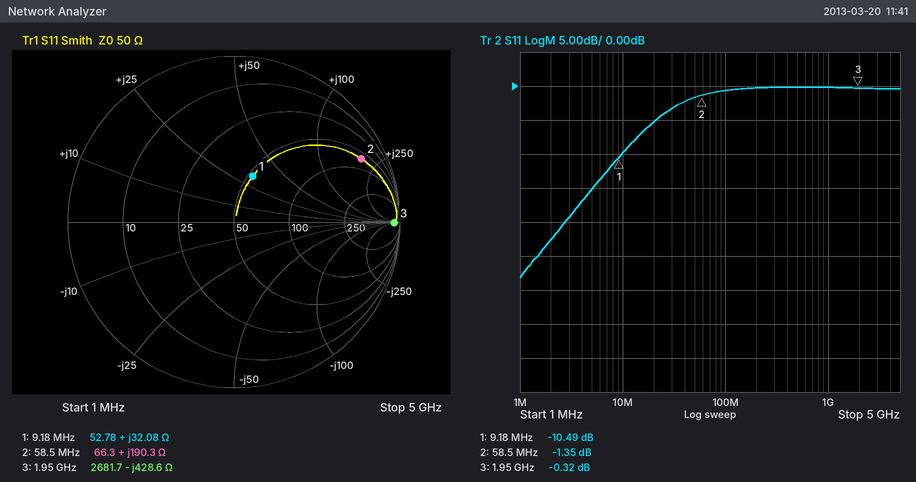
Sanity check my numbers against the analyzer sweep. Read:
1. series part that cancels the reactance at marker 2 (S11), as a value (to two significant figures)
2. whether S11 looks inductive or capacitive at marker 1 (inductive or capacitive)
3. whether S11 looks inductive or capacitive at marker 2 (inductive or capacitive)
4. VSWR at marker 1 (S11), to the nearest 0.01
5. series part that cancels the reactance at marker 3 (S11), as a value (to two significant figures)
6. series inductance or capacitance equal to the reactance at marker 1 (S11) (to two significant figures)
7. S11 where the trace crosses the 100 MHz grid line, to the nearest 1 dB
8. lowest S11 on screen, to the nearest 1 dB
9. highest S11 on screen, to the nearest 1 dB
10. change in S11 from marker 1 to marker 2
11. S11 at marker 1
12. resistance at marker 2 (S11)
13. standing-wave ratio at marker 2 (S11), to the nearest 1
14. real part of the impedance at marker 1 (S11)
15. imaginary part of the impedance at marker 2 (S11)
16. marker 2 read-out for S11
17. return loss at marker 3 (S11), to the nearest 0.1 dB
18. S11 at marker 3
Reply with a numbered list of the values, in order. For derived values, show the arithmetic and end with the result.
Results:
1. C = 1/(2π × 58.5 MHz × 190.3 Ω) ≈ 14 pF
2. inductive
3. inductive
4. 1.85
5. L = 428.6 Ω/(2π × 1.95 GHz) ≈ 35 nH
6. L = 32.08 Ω/(2π × 9.18 MHz) ≈ 556 nH, so 560 nH to two significant figures
7. -1 dB
8. -28 dB
9. 0 dB
10. -1.35 − (-10.49) = 9.14 dB
11. -10.49 dB
12. 66.3 Ω
13. 13
14. 52.78 Ω
15. +190.3 Ω
16. -1.35 dB
17. 0.3 dB
18. -0.32 dB
